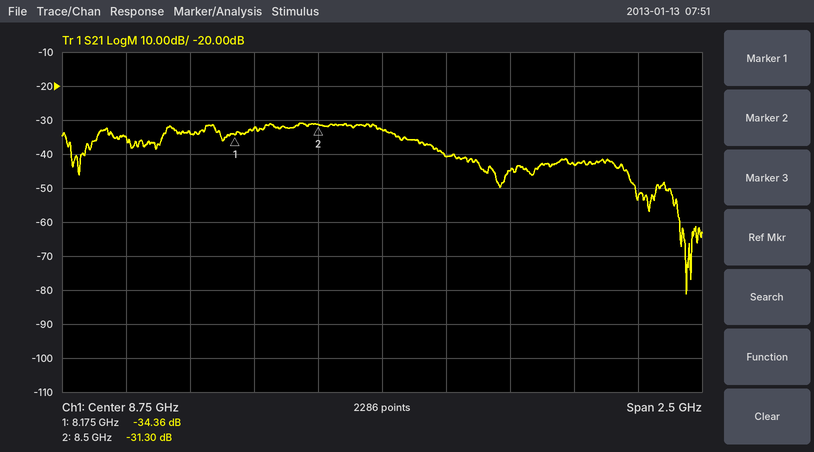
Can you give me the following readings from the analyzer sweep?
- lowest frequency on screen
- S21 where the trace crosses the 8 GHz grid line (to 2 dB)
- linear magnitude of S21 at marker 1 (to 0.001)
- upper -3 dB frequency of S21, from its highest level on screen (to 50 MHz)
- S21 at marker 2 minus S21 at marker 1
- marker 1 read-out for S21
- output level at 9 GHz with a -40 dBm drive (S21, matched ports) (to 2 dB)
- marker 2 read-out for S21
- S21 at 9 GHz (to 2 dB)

7.5 GHz
-34 dB
0.019
8.80 GHz
3.06 dB
-34.36 dB
-80 dBm
-31.30 dB
-40 dB
